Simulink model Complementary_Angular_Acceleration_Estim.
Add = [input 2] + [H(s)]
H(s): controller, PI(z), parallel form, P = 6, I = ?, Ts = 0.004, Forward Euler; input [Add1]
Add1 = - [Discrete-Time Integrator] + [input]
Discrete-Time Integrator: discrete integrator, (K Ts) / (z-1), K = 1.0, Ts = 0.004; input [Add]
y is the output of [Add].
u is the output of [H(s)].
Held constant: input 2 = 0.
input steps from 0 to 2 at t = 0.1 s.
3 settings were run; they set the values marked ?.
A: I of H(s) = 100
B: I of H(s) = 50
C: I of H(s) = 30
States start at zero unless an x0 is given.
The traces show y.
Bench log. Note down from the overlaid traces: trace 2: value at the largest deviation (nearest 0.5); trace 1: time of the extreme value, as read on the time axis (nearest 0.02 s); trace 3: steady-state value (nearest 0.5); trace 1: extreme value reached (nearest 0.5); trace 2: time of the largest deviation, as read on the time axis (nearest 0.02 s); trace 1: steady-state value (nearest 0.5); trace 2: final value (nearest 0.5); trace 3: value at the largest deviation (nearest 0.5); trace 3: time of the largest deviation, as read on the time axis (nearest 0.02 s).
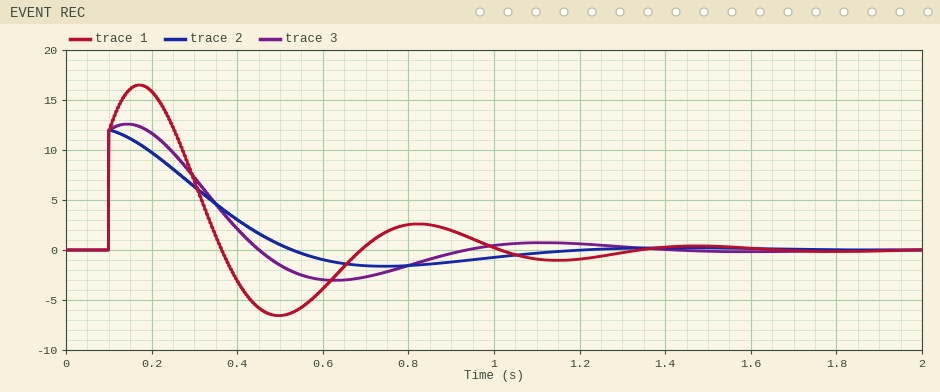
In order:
12.0
0.18 s
0.0
16.5
0.10 s
0.0
0.0
12.5
0.14 s
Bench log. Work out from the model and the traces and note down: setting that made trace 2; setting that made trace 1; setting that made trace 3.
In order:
C
A
B
